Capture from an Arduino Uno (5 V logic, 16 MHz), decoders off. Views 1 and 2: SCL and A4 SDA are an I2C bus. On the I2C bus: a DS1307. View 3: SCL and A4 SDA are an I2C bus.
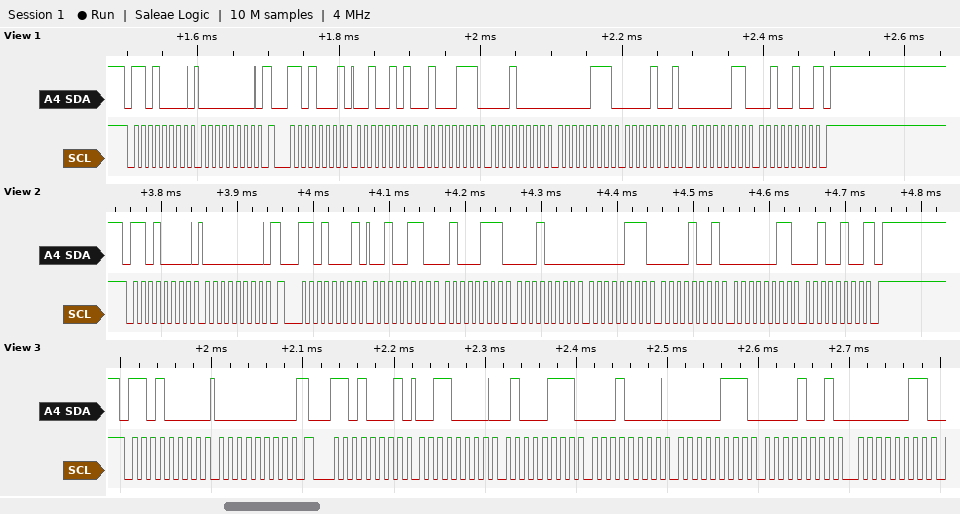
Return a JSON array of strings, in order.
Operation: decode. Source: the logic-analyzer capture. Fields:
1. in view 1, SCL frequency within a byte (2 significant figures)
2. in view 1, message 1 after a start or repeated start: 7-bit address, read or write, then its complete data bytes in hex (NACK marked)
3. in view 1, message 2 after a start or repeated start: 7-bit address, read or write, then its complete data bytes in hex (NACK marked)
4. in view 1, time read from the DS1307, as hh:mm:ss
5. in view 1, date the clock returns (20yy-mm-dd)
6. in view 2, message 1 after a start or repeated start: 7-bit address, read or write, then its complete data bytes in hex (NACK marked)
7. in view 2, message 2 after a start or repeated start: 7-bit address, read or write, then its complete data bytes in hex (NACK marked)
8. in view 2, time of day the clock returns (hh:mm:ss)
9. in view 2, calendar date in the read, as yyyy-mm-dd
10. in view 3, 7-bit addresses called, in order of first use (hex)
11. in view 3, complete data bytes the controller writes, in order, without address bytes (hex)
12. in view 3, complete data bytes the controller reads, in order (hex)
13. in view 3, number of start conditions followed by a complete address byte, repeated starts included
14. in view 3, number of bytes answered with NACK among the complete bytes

["100 kHz", "0x68 write: 00", "0x68 read: 25 47 10 07 09 03 24 NACK", "10:47:25", "2024-03-09", "0x68 write: 00", "0x68 read: 26 47 10 07 09 03 24 NACK", "10:47:26", "2024-03-09", "0x68", "00", "30 47 10 07 09 03", "2", "0"]
